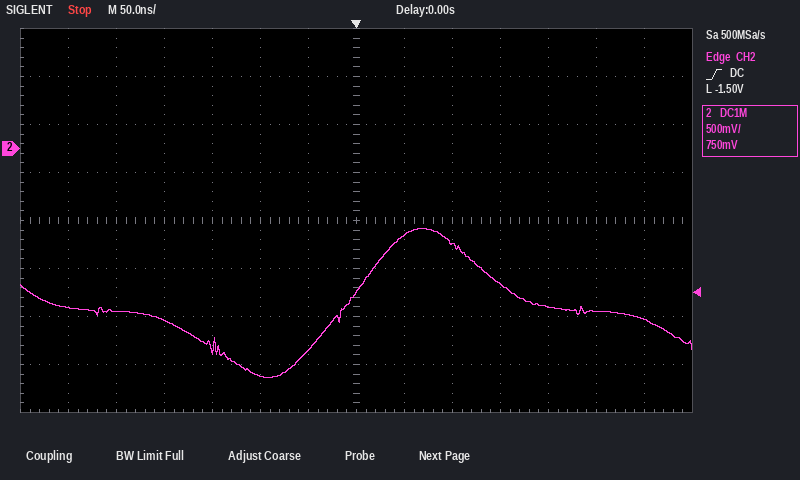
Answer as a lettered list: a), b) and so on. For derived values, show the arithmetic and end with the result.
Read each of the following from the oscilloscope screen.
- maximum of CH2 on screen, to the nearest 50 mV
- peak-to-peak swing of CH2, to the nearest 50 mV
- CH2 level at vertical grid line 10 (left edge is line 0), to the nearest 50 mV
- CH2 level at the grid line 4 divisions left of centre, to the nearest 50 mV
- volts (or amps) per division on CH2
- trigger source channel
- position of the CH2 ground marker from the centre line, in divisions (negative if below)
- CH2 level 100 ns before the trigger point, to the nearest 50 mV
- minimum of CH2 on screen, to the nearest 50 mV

a) -850 mV
b) -850 mV − (-2.40 V) = 1.55 V
c) -1.40 V
d) -1.80 V
e) 500 mV
f) CH2
g) +1.5 div
h) -2.35 V
i) -2.40 V
